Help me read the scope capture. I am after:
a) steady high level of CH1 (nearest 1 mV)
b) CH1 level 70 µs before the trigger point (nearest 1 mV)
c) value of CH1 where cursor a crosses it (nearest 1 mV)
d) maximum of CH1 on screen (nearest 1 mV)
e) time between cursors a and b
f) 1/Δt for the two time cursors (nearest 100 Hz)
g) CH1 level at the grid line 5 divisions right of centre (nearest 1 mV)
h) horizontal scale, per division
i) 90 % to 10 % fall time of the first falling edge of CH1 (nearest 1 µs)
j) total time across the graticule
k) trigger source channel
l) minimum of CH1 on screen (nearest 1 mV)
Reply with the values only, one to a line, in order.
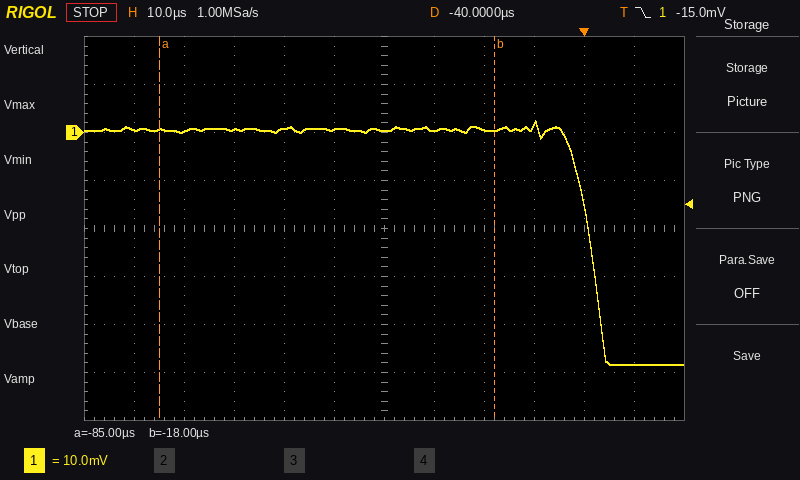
1 mV
1 mV
1 mV
2 mV
67 µs
14.9 kHz
-48 mV
10 µs
6 µs
120 µs
CH1
-48 mV
